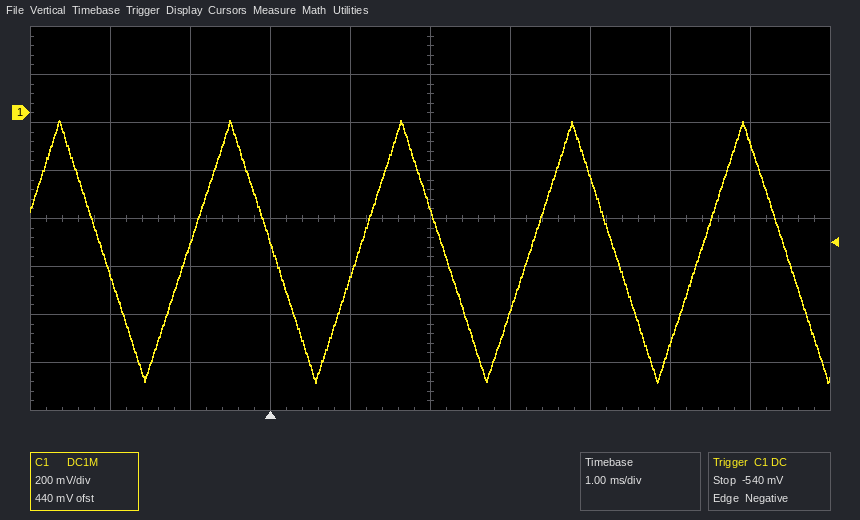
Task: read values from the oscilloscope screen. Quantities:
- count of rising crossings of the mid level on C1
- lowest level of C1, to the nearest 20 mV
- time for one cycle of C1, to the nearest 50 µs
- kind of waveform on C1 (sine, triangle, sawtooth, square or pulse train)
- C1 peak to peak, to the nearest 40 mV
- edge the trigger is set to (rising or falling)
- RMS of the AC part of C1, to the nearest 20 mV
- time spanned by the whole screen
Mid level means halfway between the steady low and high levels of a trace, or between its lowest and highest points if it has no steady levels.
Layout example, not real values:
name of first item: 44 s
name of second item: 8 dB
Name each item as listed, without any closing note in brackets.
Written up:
count of rising crossings of the mid level on C1: 4
lowest level of C1, to the nearest 20 mV: -1.12 V
time for one cycle of C1, to the nearest 50 µs: 2.15 ms
kind of waveform on C1: triangle
C1 peak to peak, to the nearest 40 mV: 1.08 V
edge the trigger is set to: falling
RMS of the AC part of C1, to the nearest 20 mV: 320 mV
time spanned by the whole screen: 10 ms
